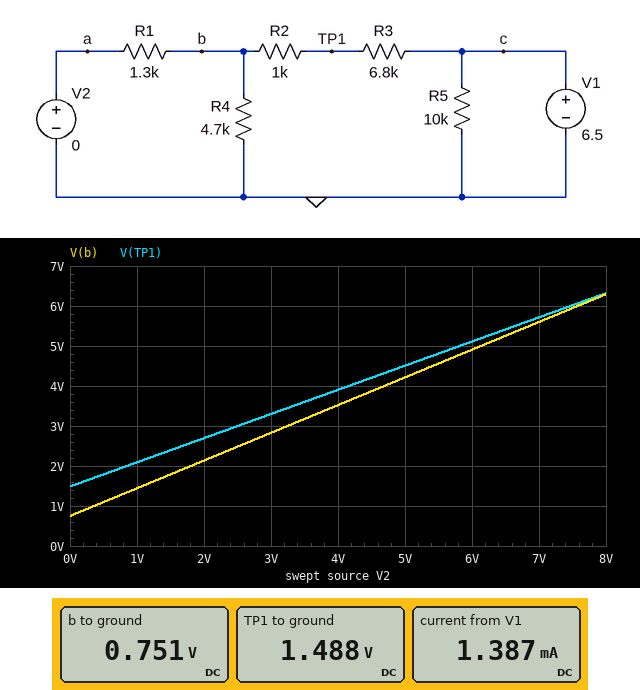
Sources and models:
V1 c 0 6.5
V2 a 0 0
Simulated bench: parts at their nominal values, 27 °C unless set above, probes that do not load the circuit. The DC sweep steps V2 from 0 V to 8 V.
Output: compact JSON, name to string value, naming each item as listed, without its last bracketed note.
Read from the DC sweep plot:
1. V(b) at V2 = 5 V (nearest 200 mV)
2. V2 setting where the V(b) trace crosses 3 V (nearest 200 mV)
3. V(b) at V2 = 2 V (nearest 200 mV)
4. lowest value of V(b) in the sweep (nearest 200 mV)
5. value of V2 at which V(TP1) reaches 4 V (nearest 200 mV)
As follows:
{"V(b) at V2 = 5 V": "4.2 V", "V2 setting where the V(b) trace crosses 3 V": "3.2 V", "V(b) at V2 = 2 V": "2.2 V", "lowest value of V(b) in the sweep": "800 mV", "value of V2 at which V(TP1) reaches 4 V": "4.2 V"}
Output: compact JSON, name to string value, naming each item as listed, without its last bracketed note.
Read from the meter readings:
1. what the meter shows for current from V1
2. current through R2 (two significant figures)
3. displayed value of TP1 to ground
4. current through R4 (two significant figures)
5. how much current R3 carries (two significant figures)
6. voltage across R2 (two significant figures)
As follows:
{"what the meter shows for current from V1": "1.387 mA", "current through R2": "740 µA", "displayed value of TP1 to ground": "1.488 V", "current through R4": "160 µA", "how much current R3 carries": "740 µA", "voltage across R2": "740 mV"}
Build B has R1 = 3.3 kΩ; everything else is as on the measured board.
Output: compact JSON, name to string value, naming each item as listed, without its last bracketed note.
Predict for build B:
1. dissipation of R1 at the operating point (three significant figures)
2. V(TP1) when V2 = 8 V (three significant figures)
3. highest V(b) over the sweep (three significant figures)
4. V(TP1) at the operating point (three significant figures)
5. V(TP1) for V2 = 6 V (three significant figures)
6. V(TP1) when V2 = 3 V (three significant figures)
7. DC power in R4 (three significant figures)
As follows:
{"dissipation of R1 at the operating point": "507 µW", "V(TP1) when V2 = 8 V": "5.24 V", "highest V(b) over the sweep": "5.06 V", "V(TP1) at the operating point": "1.96 V", "V(TP1) for V2 = 6 V": "4.42 V", "V(TP1) when V2 = 3 V": "3.19 V", "DC power in R4": "356 µW"}
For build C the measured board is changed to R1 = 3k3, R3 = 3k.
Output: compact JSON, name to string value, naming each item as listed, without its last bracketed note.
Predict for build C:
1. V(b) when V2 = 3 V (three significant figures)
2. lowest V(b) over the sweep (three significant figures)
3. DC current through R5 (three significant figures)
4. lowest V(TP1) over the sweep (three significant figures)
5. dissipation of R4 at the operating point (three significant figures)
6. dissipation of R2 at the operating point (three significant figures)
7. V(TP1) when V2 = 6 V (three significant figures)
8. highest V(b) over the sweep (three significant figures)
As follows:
{"V(b) when V2 = 3 V": "3.31 V", "lowest V(b) over the sweep": "2.12 V", "DC current through R5": "650 µA", "lowest V(TP1) over the sweep": "3.22 V", "dissipation of R4 at the operating point": "958 µW", "dissipation of R2 at the operating point": "1.20 mW", "V(TP1) when V2 = 6 V": "5.00 V", "highest V(b) over the sweep": "5.29 V"}
